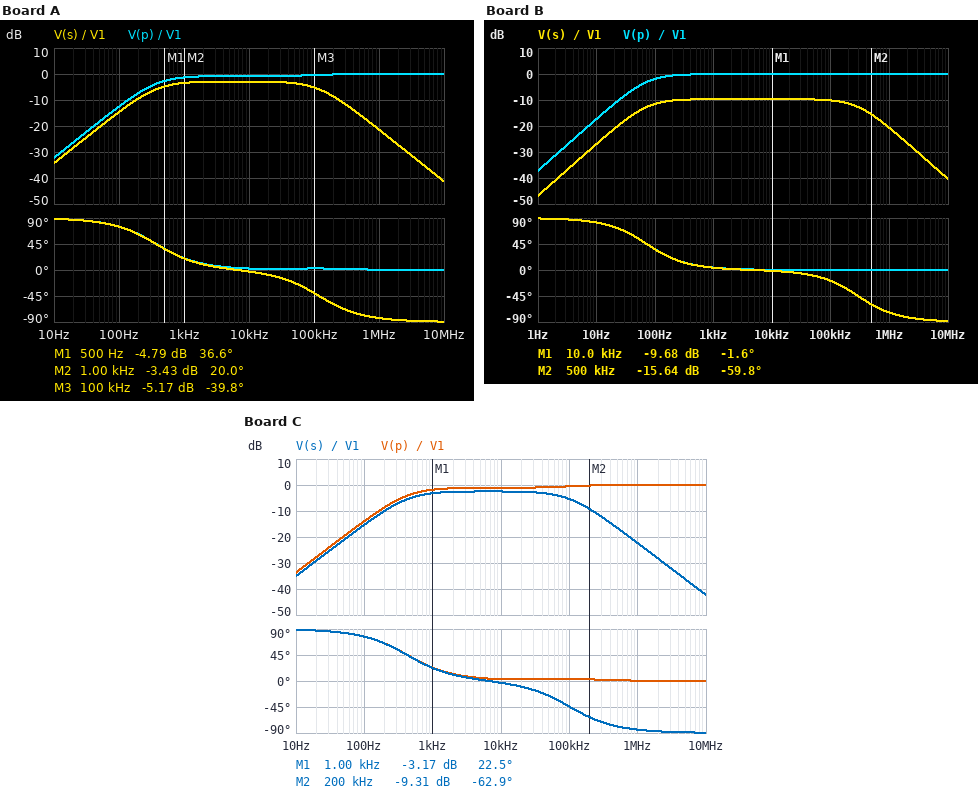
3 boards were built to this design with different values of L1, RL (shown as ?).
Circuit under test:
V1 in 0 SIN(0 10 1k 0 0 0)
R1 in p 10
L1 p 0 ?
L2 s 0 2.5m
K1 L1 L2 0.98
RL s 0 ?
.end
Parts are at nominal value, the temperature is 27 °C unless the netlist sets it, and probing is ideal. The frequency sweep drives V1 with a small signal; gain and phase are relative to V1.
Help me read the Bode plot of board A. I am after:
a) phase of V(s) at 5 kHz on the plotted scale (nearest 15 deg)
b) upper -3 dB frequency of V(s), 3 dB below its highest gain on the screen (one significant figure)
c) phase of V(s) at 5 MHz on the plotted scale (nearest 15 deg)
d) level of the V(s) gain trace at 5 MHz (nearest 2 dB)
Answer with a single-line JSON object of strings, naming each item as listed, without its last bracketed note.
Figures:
{"phase of V(s) at 5 kHz on the plotted scale": "0 deg", "upper -3 dB frequency of V(s), 3 dB below its highest gain on the screen": "100 kHz", "phase of V(s) at 5 MHz on the plotted scale": "-90 deg", "level of the V(s) gain trace at 5 MHz": "-36 dB"}
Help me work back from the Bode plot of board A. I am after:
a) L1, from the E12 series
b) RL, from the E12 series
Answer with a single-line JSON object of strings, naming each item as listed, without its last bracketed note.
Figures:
{"L1, from the E12 series": "3.9 mH", "RL, from the E12 series": "68 Ω"}
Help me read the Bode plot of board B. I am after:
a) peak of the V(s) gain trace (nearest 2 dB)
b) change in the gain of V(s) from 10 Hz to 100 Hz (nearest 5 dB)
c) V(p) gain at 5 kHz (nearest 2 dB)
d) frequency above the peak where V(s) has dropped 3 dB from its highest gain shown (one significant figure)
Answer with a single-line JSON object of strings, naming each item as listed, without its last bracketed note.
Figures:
{"peak of the V(s) gain trace": "-10 dB", "change in the gain of V(s) from 10 Hz to 100 Hz": "15 dB", "V(p) gain at 5 kHz": "0 dB", "frequency above the peak where V(s) has dropped 3 dB from its highest gain shown": "300 kHz"}
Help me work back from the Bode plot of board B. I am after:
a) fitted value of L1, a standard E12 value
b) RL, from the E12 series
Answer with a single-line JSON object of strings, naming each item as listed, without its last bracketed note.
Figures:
{"fitted value of L1, a standard E12 value": "22 mH", "RL, from the E12 series": "180 Ω"}
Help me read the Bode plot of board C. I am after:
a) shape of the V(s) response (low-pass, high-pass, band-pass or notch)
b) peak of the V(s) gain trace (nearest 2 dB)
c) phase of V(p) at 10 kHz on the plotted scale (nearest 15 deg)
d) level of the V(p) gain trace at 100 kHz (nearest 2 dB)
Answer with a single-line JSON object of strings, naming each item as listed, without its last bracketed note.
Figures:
{"shape of the V(s) response": "band-pass", "peak of the V(s) gain trace": "-2 dB", "phase of V(p) at 10 kHz on the plotted scale": "0 deg", "level of the V(p) gain trace at 100 kHz": "0 dB"}
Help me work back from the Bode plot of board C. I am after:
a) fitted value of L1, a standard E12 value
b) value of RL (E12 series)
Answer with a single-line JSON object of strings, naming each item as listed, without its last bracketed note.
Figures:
{"fitted value of L1, a standard E12 value": "3.3 mH", "value of RL": "56 Ω"}
